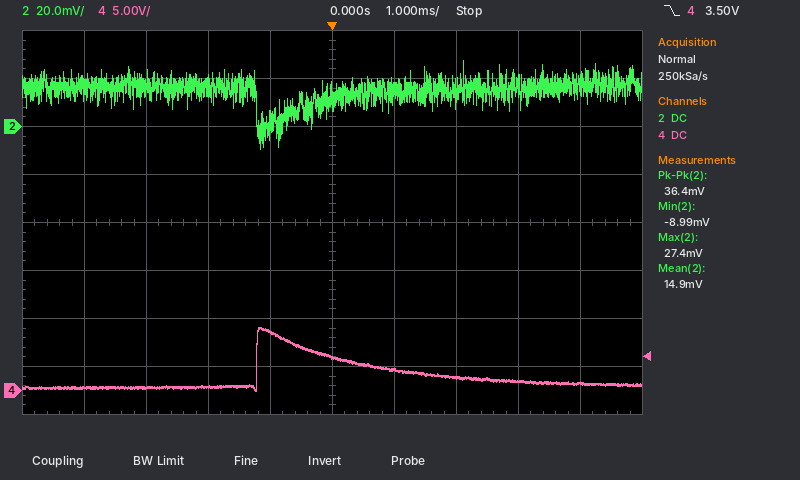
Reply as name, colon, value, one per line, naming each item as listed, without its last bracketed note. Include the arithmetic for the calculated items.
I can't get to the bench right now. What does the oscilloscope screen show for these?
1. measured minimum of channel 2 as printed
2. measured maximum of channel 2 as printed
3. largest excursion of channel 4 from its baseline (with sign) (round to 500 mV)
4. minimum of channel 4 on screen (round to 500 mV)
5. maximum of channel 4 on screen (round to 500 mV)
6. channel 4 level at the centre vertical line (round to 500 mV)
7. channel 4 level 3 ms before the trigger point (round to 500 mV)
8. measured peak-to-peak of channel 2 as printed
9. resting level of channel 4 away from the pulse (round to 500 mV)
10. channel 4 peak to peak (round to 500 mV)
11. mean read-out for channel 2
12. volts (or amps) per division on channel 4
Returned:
measured minimum of channel 2 as printed: -8.99 mV
measured maximum of channel 2 as printed: 27.4 mV
largest excursion of channel 4 from its baseline (with sign): 6.5 V − (500 mV) = +6.0 V
minimum of channel 4 on screen: 0.0 V
maximum of channel 4 on screen: 6.5 V
channel 4 level at the centre vertical line: 3.5 V
channel 4 level 3 ms before the trigger point: 500 mV
measured peak-to-peak of channel 2 as printed: 36.4 mV
resting level of channel 4 away from the pulse: 500 mV
channel 4 peak to peak: 6.5 V − (0.0 V) = 6.5 V
mean read-out for channel 2: 14.9 mV
volts (or amps) per division on channel 4: 5 V
